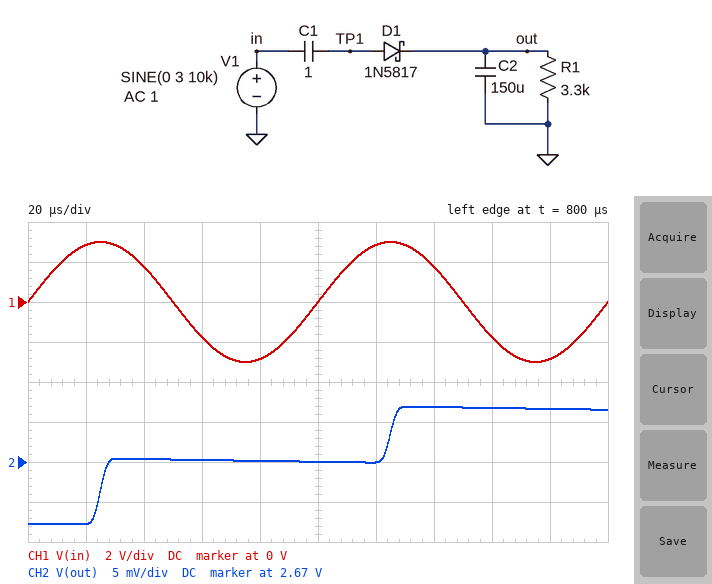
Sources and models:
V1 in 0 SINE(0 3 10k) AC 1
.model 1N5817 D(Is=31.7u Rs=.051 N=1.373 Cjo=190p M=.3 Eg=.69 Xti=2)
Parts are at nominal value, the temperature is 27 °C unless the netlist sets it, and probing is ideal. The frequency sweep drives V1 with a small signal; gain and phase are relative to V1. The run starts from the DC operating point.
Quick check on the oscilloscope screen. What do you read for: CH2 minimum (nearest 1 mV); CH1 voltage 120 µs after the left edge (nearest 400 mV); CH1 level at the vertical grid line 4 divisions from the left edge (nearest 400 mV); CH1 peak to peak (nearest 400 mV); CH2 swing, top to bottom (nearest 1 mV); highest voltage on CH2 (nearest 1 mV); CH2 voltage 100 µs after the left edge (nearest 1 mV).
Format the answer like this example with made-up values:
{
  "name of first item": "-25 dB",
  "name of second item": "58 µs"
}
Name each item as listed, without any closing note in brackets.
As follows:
{
  "CH2 minimum": "2.662 V",
  "CH1 voltage 120 µs after the left edge": "2.8 V",
  "CH1 level at the vertical grid line 4 divisions from the left edge": "-2.8 V",
  "CH1 peak to peak": "6.0 V",
  "CH2 swing, top to bottom": "15 mV",
  "highest voltage on CH2": "2.677 V",
  "CH2 voltage 100 µs after the left edge": "2.670 V"
}
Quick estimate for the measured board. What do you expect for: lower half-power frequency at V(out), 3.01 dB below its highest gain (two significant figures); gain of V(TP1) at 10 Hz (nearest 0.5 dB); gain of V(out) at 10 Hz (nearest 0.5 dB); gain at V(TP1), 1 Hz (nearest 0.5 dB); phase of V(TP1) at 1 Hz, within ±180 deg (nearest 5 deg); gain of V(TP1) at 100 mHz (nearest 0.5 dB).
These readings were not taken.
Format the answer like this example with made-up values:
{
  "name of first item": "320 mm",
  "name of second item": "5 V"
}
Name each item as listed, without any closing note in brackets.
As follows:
{
  "lower half-power frequency at V(out), 3.01 dB below its highest gain": "36 µHz",
  "gain of V(TP1) at 10 Hz": "0 dB",
  "gain of V(out) at 10 Hz": "-20.5 dB",
  "gain at V(TP1), 1 Hz": "0 dB",
  "phase of V(TP1) at 1 Hz, within ±180 deg": "0 deg",
  "gain of V(TP1) at 100 mHz": "0 dB"
}
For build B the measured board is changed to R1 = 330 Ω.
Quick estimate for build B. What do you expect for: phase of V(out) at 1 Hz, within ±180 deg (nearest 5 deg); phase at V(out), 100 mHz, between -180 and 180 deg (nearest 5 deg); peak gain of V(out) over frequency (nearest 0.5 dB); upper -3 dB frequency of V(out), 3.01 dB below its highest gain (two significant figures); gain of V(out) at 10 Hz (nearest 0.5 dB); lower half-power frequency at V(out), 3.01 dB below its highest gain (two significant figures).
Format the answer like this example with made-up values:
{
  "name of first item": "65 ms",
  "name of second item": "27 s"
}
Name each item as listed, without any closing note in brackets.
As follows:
{
  "phase of V(out) at 1 Hz, within ±180 deg": "-15 deg",
  "phase at V(out), 100 mHz, between -180 and 180 deg": "0 deg",
  "peak gain of V(out) over frequency": "-13.0 dB",
  "upper -3 dB frequency of V(out), 3.01 dB below its highest gain": "4.2 Hz",
  "gain of V(out) at 10 Hz": "-21.0 dB",
  "lower half-power frequency at V(out), 3.01 dB below its highest gain": "110 µHz"
}
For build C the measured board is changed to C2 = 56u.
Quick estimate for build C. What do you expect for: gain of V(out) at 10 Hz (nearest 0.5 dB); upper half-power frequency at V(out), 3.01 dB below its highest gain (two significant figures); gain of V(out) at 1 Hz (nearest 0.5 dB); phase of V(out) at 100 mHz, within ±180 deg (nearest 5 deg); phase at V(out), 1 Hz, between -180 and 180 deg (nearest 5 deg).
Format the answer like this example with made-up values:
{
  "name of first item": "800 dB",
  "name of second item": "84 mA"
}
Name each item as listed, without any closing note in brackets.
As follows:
{
  "gain of V(out) at 10 Hz": "-12.5 dB",
  "upper half-power frequency at V(out), 3.01 dB below its highest gain": "3.4 Hz",
  "gain of V(out) at 1 Hz": "-3.0 dB",
  "phase of V(out) at 100 mHz, within ±180 deg": "0 deg",
  "phase at V(out), 1 Hz, between -180 and 180 deg": "-15 deg"
}
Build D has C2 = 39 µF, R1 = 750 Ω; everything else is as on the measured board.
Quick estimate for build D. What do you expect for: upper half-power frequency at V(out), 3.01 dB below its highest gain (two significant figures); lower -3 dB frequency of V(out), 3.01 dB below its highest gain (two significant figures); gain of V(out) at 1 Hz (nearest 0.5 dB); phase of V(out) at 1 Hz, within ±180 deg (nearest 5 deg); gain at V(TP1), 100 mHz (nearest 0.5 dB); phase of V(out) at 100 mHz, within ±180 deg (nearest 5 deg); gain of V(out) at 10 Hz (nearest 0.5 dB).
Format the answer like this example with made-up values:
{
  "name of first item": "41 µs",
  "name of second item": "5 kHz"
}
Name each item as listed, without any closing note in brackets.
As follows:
{
  "upper half-power frequency at V(out), 3.01 dB below its highest gain": "9.1 Hz",
  "lower -3 dB frequency of V(out), 3.01 dB below its highest gain": "85 µHz",
  "gain of V(out) at 1 Hz": "-8.0 dB",
  "phase of V(out) at 1 Hz, within ±180 deg": "-5 deg",
  "gain at V(TP1), 100 mHz": "0 dB",
  "phase of V(out) at 100 mHz, within ±180 deg": "0 deg",
  "gain of V(out) at 10 Hz": "-11.5 dB"
}
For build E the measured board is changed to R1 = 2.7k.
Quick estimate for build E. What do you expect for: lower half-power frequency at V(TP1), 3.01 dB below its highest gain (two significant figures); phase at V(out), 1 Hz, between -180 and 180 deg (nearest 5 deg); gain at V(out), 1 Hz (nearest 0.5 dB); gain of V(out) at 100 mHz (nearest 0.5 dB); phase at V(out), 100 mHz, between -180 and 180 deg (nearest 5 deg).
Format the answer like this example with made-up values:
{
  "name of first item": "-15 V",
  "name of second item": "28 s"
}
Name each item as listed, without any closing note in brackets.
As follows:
{
  "lower half-power frequency at V(TP1), 3.01 dB below its highest gain": "42 µHz",
  "phase at V(out), 1 Hz, between -180 and 180 deg": "-35 deg",
  "gain at V(out), 1 Hz": "-5.0 dB",
  "gain of V(out) at 100 mHz": "-3.0 dB",
  "phase at V(out), 100 mHz, between -180 and 180 deg": "-5 deg"
}
